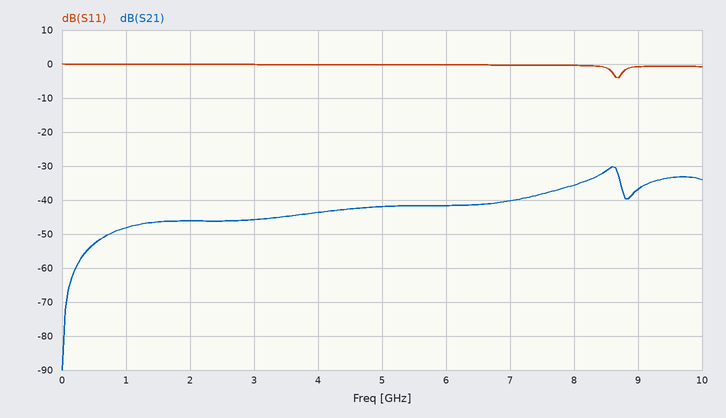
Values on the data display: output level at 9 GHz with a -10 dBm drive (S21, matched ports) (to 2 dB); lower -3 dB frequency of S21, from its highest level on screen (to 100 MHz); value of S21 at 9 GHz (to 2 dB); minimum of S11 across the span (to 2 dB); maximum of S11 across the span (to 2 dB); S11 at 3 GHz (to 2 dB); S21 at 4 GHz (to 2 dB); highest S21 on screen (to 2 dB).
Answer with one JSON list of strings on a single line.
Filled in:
["-46 dBm", "8.3 GHz", "-36 dB", "-4 dB", "0 dB", "0 dB", "-44 dB", "-30 dB"]
